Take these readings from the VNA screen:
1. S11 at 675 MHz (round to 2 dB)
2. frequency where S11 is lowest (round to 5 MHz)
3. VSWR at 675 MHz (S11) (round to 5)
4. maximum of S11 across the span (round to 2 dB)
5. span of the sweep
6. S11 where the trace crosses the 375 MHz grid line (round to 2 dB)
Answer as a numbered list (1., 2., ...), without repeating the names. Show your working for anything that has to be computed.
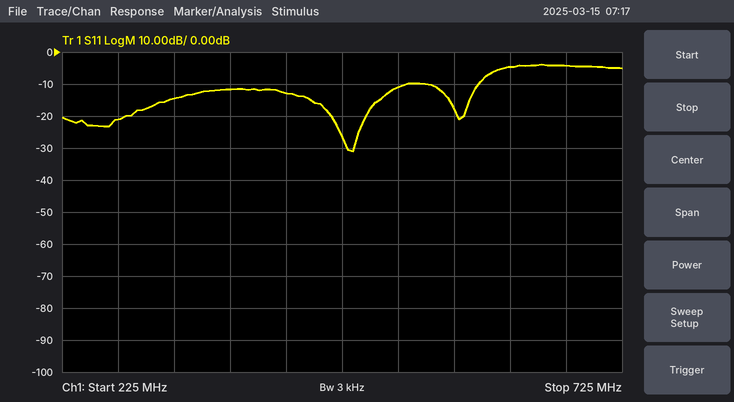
1. -4 dB
2. 485 MHz
3. |Γ| = 10^(-4/20) = 0.6310; VSWR = (1 + 0.6310)/(1 − 0.6310) ≈ 4.42, so 5 to the nearest 5
4. -4 dB
5. 500 MHz
6. -12 dB
